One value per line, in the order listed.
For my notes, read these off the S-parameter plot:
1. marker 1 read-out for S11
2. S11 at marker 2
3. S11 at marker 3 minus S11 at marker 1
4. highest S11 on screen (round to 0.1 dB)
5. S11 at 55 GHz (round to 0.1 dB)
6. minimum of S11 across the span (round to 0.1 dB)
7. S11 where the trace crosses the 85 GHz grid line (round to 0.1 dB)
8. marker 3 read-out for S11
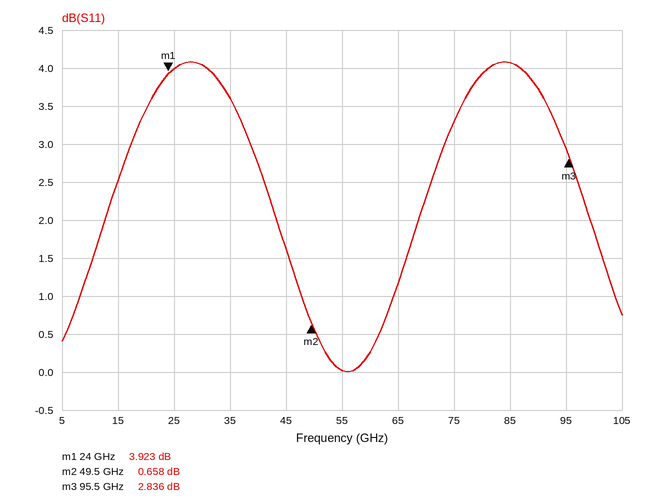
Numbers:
3.923 dB
0.658 dB
-1.087 dB
4.1 dB
0.0 dB
0.0 dB
4.1 dB
2.836 dB
